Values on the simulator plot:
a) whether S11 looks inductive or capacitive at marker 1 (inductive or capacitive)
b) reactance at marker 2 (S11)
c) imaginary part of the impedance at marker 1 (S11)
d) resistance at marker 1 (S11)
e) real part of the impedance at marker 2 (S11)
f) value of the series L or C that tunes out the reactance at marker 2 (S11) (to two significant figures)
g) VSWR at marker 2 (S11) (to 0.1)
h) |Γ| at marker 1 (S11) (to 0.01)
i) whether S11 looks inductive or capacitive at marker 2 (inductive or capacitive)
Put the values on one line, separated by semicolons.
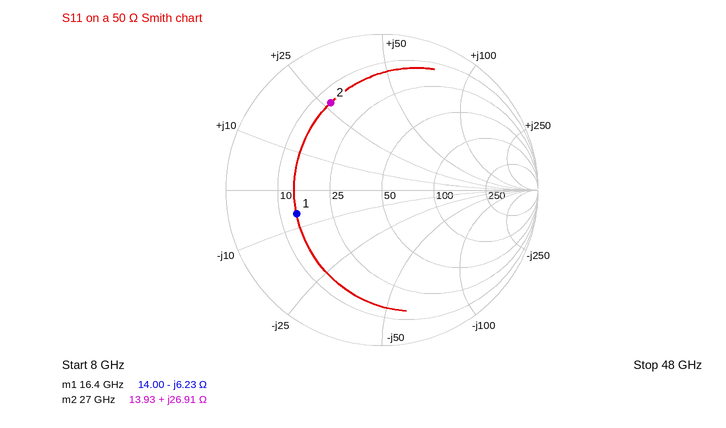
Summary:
capacitive; +26.91 Ω; -6.23 Ω; 14.00 Ω; 13.93 Ω; 220 fF; 4.7; 0.57; inductive
